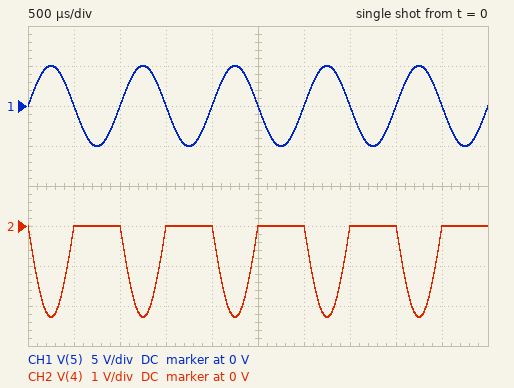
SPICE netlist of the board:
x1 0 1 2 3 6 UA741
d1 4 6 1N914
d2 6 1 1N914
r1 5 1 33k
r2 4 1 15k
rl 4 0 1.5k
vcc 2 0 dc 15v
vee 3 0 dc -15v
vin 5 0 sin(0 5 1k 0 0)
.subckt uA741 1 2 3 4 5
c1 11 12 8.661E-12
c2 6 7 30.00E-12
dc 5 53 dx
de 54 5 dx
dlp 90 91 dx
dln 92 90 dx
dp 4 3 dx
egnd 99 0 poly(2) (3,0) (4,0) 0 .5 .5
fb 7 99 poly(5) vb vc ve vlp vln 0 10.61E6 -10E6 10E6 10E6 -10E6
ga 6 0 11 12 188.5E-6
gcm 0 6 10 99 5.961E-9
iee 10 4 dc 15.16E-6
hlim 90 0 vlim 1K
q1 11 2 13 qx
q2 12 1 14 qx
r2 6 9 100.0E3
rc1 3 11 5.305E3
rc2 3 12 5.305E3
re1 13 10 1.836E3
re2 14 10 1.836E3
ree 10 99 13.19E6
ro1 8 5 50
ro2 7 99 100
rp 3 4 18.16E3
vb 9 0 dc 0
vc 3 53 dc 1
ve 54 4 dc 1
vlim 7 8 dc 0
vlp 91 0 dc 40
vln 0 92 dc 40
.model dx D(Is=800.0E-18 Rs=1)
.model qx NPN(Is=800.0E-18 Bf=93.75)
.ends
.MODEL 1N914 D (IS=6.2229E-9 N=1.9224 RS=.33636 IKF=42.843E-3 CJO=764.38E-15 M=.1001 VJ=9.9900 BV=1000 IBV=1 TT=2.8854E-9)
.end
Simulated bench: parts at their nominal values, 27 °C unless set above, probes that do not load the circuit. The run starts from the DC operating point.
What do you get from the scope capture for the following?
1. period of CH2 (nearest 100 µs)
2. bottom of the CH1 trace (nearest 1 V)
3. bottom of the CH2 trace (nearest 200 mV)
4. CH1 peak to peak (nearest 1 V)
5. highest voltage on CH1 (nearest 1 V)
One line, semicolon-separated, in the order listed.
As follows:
1.0 ms; -5 V; -2.2 V; 10 V; 5 V
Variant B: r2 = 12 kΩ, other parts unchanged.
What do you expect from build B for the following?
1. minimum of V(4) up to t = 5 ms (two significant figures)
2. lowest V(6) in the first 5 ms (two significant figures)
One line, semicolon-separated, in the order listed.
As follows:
-1.8 V; -2.4 V
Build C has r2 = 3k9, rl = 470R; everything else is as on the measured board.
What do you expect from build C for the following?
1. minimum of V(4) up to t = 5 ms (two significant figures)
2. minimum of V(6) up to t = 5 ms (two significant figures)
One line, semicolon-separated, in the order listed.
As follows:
-590 mV; -1.2 V
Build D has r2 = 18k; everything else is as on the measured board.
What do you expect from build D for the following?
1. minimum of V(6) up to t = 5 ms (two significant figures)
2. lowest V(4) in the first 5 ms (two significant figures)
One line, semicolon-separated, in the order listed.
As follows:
-3.4 V; -2.7 V
